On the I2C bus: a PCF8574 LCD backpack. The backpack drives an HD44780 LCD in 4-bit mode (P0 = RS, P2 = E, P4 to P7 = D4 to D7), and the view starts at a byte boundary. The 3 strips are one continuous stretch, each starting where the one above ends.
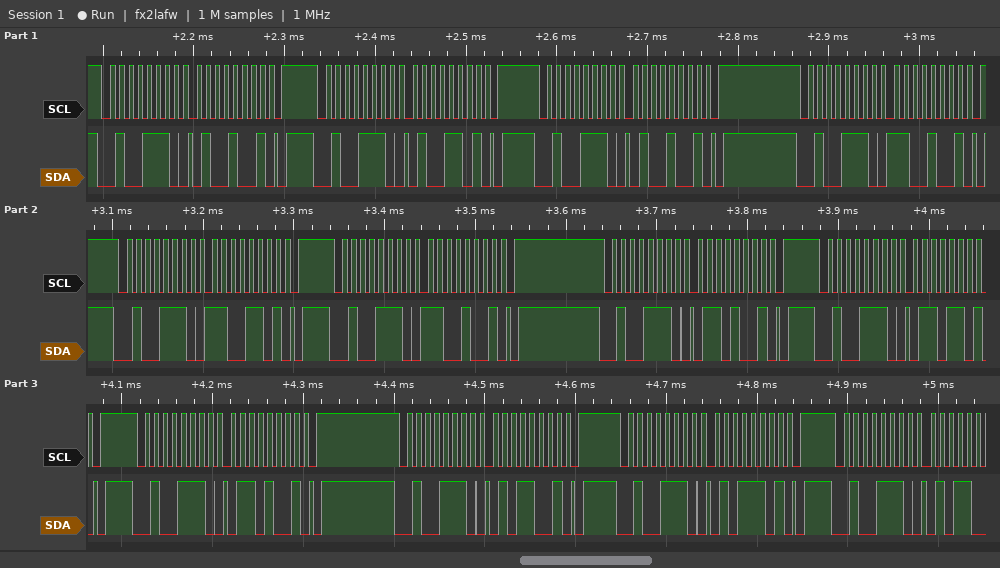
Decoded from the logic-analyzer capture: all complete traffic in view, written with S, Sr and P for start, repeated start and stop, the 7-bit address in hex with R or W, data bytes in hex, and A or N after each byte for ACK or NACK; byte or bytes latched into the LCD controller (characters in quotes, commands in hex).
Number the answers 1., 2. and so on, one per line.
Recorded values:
1. S 27W A 49 A P S 27W A 4D A P S 27W A 49 A P S 27W A C9 A P S 27W A CD A P S 27W A C9 A P S 27W A 69 A P S 27W A 6D A P S 27W A 69 A P S 27W A 59 A P S 27W A 5D A P S 27W A
2. 'L'
